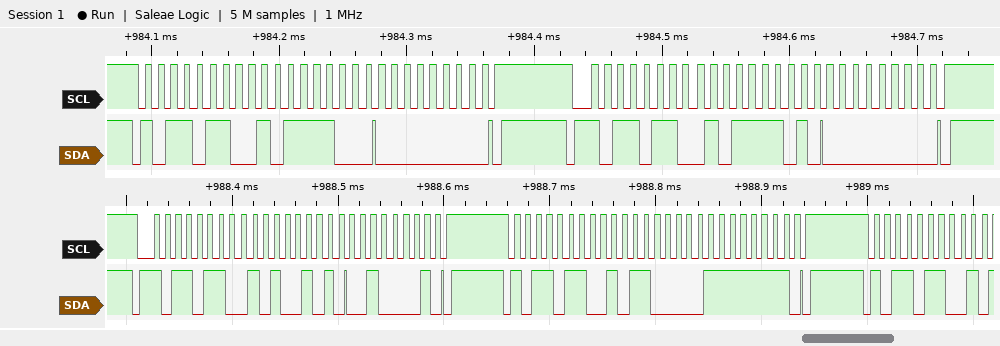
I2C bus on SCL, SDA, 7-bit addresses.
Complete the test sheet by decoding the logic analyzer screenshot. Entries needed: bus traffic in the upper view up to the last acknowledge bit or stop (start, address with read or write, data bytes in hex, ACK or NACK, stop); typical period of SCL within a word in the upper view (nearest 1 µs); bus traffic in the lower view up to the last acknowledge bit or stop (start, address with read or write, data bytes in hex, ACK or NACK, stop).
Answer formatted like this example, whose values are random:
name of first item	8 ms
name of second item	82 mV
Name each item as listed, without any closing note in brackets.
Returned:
bus traffic in the upper view up to the last acknowledge bit or stop	start, address 5B write ACK, BC ACK, 00 ACK, stop, start, address 5B write ACK, BD ACK, 00 ACK, stop
typical period of SCL within a word in the upper view	10 µs
bus traffic in the lower view up to the last acknowledge bit or stop	start, address 5B write ACK, A5 ACK, 21 ACK, stop, start, address 5B write ACK, B0 ACK, FF ACK, stop, start, address 5B write ACK
